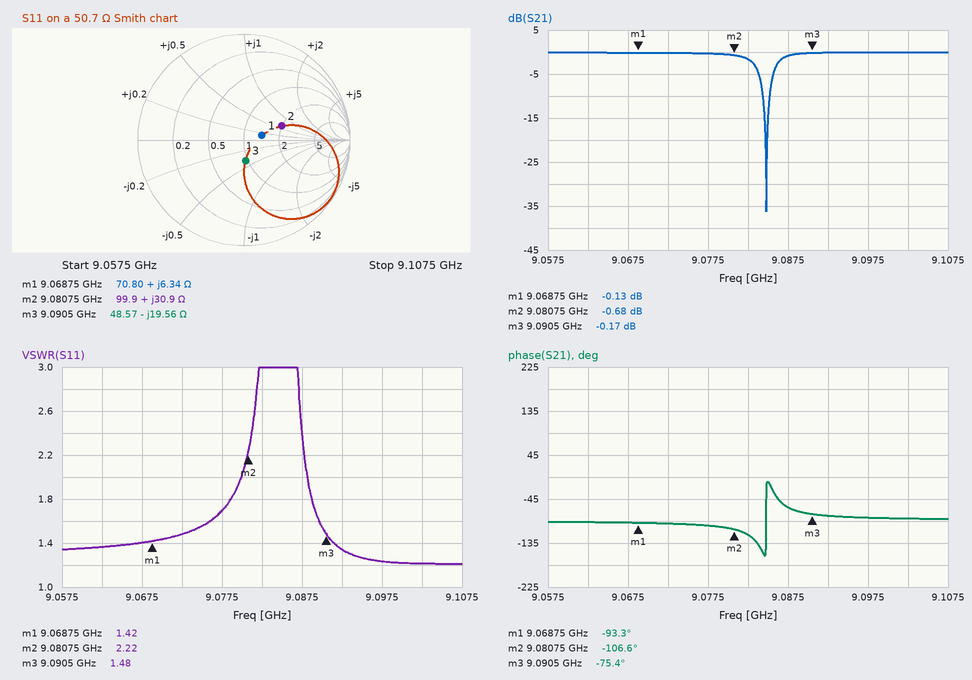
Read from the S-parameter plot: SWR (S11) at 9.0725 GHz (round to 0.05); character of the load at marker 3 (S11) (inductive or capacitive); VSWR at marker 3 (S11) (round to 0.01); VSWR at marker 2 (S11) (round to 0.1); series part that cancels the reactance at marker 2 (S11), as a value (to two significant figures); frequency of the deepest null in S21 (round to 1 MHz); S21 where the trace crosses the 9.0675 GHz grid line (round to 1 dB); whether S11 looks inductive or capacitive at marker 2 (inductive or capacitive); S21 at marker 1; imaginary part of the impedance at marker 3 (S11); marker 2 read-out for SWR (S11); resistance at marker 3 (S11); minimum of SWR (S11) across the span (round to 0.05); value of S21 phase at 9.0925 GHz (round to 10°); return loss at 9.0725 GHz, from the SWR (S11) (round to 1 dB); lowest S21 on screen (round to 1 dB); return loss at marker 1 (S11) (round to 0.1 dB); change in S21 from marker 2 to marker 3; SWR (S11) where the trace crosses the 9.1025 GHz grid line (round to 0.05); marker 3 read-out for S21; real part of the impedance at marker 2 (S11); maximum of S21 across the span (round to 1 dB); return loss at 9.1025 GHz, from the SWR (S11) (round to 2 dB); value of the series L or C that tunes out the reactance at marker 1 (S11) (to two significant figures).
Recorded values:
1.50
capacitive
1.48
2.2
570 fF
9.085 GHz
0 dB
inductive
-0.13 dB
-19.56 Ω
2.22
48.57 Ω
1.20
-80°
14 dB
-36 dB
15.2 dB
0.51 dB
1.20
-0.17 dB
99.9 Ω
0 dB
20 dB
2.8 pF
